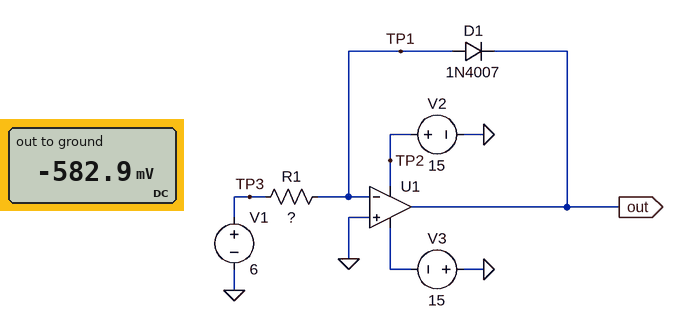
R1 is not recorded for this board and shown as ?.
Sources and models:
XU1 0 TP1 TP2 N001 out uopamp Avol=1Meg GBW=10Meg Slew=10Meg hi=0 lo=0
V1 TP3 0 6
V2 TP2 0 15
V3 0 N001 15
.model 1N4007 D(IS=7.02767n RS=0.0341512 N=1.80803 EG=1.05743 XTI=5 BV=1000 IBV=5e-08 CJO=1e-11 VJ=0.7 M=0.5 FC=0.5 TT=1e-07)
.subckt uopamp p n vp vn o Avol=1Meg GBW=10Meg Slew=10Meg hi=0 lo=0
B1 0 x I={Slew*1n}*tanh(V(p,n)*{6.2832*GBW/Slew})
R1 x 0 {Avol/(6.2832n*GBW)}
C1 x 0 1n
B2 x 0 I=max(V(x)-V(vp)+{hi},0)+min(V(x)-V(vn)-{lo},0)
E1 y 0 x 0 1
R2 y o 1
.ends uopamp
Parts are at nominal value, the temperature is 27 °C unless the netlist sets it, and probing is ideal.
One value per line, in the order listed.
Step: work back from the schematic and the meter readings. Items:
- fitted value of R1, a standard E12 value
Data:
3.3 kΩ
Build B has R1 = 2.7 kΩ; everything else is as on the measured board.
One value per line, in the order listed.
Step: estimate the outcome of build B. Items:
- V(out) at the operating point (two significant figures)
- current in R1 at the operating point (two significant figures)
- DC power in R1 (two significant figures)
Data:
-590 mV
2.2 mA
13 mW
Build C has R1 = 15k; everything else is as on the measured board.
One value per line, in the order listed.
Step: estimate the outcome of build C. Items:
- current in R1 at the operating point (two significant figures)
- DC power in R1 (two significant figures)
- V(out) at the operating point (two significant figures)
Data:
400 µA
2.4 mW
-510 mV
